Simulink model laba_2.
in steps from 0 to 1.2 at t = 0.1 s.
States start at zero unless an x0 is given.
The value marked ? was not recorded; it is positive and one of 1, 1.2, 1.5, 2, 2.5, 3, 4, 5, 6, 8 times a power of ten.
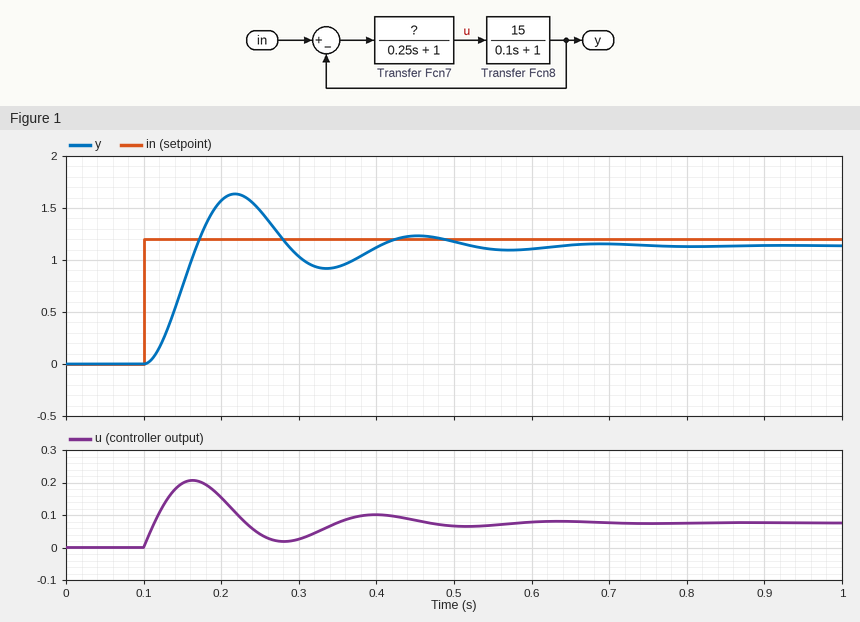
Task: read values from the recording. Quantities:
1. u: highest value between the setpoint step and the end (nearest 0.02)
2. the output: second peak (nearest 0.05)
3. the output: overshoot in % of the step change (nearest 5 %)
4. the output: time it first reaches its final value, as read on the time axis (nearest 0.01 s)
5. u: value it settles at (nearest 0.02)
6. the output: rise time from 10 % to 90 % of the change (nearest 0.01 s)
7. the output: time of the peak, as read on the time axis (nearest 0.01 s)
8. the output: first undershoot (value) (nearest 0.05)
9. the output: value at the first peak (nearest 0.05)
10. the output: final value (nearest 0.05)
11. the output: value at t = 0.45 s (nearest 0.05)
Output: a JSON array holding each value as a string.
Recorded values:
["0.20", "1.25", "45 %", "0.17 s", "0.08", "0.05 s", "0.22 s", "0.90", "1.65", "1.15", "1.25"]
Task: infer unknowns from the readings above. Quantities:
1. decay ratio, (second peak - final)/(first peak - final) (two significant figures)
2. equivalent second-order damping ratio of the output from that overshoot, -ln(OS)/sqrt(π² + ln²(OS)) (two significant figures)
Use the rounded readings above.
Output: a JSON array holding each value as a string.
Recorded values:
["0.20", "0.25"]
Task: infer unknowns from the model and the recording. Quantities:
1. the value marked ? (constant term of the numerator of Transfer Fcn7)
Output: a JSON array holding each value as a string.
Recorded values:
["1.2"]
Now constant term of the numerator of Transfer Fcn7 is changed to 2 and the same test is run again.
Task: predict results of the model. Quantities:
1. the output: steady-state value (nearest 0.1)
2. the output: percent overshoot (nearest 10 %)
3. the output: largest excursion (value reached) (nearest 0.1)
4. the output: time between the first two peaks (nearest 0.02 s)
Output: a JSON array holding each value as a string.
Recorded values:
["1.2", "50 %", "1.8", "0.18 s"]
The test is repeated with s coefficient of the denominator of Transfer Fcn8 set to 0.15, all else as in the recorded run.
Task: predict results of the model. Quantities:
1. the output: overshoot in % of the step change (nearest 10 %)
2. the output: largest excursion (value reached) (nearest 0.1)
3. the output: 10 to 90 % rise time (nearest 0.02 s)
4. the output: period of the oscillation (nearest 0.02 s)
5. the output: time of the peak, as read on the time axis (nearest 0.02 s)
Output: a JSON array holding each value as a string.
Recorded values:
["50 %", "1.7", "0.06 s", "0.28 s", "0.24 s"]
